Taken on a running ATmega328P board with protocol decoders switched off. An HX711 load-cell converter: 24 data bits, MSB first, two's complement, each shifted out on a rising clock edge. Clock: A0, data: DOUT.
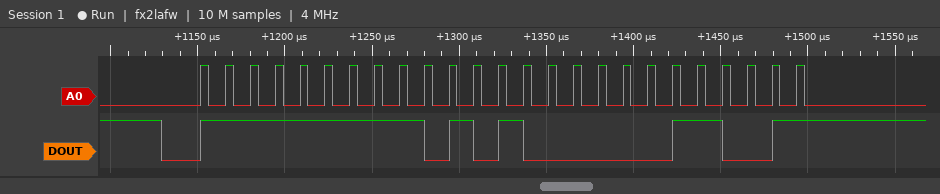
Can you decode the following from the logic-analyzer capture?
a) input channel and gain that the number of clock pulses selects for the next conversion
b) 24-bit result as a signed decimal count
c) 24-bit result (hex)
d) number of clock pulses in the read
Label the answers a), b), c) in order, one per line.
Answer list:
a) channel A, gain 128
b) -22503
c) 0xFFA819
d) 25
